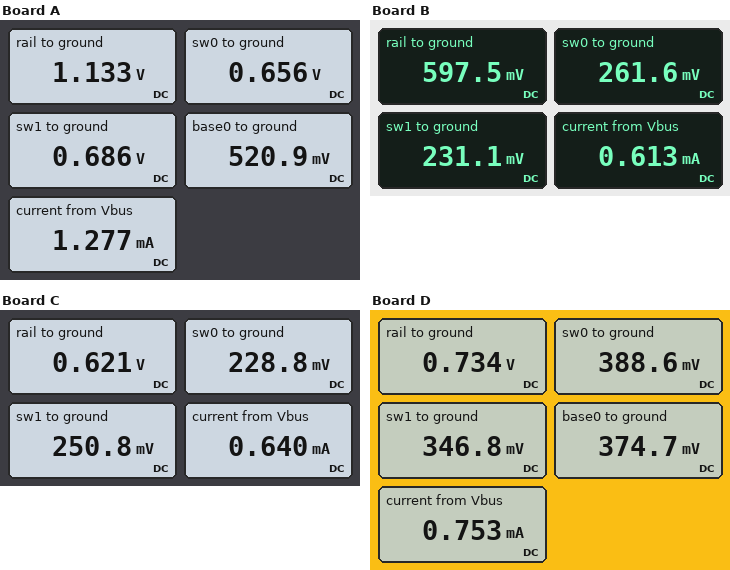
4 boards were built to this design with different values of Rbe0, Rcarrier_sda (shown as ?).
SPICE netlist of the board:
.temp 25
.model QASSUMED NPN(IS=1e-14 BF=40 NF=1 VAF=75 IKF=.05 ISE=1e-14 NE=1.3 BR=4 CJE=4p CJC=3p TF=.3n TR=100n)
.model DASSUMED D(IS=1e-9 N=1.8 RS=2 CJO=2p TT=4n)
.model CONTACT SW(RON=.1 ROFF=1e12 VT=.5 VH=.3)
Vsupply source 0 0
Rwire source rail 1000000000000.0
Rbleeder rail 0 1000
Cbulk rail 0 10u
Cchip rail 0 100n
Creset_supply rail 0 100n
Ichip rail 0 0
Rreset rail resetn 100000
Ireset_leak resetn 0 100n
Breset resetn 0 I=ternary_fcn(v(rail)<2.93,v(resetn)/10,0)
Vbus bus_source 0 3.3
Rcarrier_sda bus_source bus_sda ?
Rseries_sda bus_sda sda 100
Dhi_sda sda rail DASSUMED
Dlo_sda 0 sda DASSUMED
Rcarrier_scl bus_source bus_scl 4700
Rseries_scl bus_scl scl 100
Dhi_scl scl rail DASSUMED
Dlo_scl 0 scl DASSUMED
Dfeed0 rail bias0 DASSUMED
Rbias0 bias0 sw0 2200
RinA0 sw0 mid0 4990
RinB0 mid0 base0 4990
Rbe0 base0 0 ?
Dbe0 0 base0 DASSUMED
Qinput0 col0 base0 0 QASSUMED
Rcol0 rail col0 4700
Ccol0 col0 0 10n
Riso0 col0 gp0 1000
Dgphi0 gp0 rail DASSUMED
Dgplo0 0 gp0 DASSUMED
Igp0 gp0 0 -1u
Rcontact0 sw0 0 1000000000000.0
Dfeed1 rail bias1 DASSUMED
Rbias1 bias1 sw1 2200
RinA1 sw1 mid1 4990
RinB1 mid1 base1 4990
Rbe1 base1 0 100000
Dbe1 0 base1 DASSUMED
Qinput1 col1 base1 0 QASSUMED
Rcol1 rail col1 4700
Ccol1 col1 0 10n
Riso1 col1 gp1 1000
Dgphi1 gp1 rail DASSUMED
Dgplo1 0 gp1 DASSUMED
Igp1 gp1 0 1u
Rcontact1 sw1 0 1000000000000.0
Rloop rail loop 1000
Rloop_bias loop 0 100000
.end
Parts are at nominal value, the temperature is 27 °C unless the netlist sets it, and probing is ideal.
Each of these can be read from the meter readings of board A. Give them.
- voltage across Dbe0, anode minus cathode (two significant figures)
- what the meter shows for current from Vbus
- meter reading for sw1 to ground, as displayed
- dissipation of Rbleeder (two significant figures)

-520 mV
1.277 mA
0.686 V
1.3 mW
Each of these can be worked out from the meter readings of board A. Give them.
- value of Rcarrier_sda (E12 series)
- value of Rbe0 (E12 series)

1.5 kΩ
39 kΩ
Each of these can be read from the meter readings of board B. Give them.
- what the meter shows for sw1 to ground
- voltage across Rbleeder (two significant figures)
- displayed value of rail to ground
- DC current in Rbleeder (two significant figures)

231.1 mV
600 mV
597.5 mV
600 µA
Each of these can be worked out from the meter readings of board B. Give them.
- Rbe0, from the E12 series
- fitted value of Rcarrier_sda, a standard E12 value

220 kΩ
12 kΩ
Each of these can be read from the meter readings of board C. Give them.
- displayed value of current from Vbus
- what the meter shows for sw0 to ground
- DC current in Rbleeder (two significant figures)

0.640 mA
228.8 mV
620 µA
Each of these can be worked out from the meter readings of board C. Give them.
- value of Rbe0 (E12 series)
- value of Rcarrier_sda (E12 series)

56 kΩ
10 kΩ
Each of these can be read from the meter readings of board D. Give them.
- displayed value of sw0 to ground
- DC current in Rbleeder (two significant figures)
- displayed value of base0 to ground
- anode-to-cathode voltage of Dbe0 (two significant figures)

388.6 mV
730 µA
374.7 mV
-370 mV
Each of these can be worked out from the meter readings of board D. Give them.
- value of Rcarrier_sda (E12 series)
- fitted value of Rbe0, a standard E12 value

5.6 kΩ
270 kΩ
